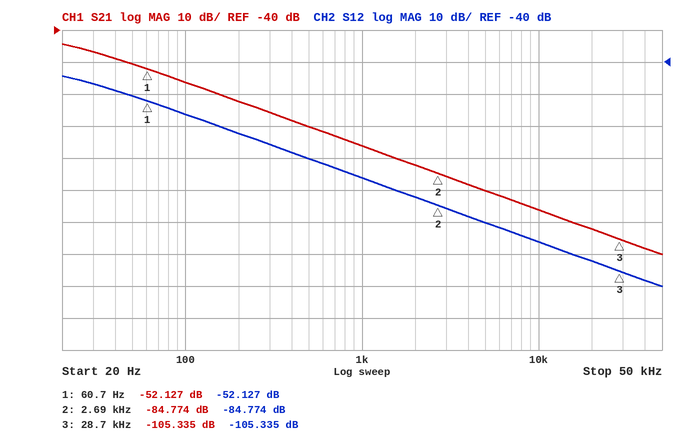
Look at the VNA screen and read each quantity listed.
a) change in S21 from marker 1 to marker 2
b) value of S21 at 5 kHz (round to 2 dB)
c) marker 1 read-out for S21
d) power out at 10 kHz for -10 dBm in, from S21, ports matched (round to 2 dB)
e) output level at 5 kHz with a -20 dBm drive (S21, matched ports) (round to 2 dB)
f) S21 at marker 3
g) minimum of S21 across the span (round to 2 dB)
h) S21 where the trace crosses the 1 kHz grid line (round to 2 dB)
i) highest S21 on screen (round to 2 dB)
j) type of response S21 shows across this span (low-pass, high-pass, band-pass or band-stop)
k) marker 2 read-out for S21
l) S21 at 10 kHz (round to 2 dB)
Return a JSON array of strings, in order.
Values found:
["-32.647 dB", "-90 dB", "-52.127 dB", "-106 dBm", "-110 dBm", "-105.335 dB", "-110 dB", "-76 dB", "-44 dB", "low-pass", "-84.774 dB", "-96 dB"]
